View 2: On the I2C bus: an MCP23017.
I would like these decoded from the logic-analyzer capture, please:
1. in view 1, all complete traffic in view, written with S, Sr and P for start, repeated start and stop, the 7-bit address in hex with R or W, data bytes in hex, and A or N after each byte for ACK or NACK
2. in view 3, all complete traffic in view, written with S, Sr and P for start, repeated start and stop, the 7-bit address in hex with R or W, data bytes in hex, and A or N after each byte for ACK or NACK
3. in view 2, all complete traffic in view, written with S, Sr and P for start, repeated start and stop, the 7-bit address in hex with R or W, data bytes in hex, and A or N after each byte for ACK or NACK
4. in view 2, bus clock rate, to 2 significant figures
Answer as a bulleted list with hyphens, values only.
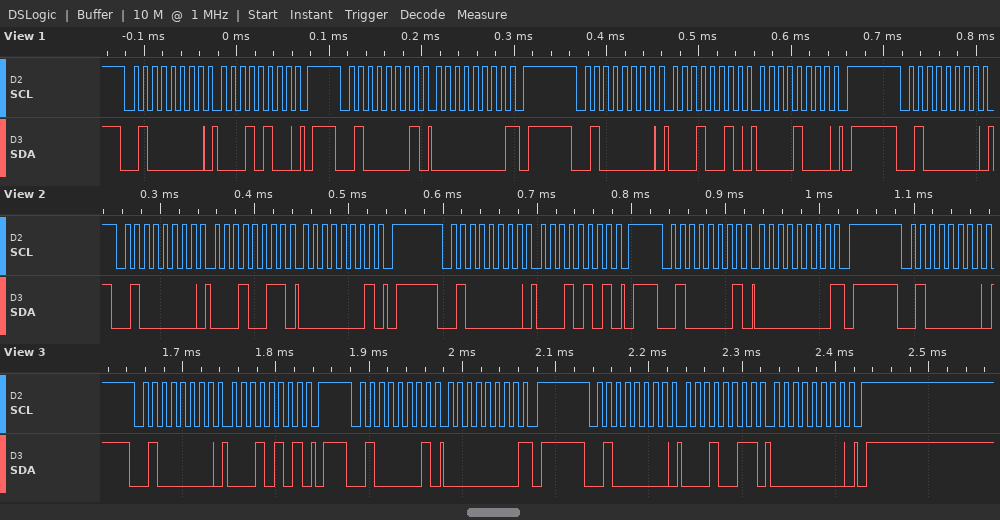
- S 20W A 14 A P S 20R A 00 N P S 20W A 12 A 08 A P S 20W A
- S 20W A 15 A P S 20R A 00 N P S 20W A 13 A 00 A P
- S 20W A 13 A 01 A P S 20W A 15 A P S 20R A 00 N P S 20W A
- 100 kHz
